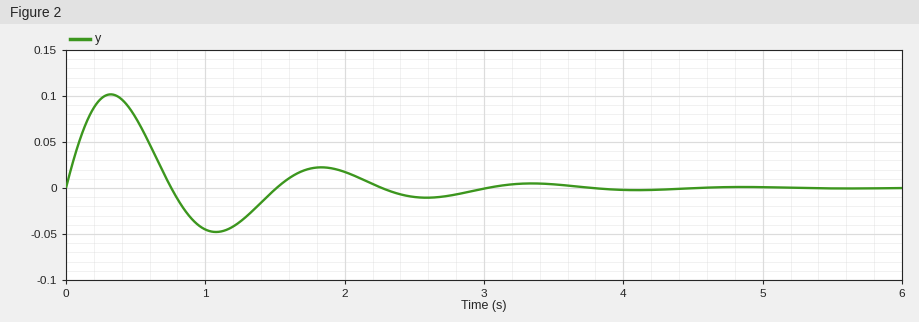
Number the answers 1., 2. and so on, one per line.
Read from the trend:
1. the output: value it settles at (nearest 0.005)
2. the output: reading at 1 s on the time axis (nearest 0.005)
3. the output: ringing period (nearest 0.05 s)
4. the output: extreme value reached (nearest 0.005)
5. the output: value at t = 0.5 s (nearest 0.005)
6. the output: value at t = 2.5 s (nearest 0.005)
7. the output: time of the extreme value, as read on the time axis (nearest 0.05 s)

1. 0.000
2. -0.045
3. 1.50 s
4. 0.100
5. 0.075
6. -0.010
7. 0.30 s
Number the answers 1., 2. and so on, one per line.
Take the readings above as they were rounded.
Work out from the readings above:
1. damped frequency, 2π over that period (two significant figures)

1. 4.2 rad/s
